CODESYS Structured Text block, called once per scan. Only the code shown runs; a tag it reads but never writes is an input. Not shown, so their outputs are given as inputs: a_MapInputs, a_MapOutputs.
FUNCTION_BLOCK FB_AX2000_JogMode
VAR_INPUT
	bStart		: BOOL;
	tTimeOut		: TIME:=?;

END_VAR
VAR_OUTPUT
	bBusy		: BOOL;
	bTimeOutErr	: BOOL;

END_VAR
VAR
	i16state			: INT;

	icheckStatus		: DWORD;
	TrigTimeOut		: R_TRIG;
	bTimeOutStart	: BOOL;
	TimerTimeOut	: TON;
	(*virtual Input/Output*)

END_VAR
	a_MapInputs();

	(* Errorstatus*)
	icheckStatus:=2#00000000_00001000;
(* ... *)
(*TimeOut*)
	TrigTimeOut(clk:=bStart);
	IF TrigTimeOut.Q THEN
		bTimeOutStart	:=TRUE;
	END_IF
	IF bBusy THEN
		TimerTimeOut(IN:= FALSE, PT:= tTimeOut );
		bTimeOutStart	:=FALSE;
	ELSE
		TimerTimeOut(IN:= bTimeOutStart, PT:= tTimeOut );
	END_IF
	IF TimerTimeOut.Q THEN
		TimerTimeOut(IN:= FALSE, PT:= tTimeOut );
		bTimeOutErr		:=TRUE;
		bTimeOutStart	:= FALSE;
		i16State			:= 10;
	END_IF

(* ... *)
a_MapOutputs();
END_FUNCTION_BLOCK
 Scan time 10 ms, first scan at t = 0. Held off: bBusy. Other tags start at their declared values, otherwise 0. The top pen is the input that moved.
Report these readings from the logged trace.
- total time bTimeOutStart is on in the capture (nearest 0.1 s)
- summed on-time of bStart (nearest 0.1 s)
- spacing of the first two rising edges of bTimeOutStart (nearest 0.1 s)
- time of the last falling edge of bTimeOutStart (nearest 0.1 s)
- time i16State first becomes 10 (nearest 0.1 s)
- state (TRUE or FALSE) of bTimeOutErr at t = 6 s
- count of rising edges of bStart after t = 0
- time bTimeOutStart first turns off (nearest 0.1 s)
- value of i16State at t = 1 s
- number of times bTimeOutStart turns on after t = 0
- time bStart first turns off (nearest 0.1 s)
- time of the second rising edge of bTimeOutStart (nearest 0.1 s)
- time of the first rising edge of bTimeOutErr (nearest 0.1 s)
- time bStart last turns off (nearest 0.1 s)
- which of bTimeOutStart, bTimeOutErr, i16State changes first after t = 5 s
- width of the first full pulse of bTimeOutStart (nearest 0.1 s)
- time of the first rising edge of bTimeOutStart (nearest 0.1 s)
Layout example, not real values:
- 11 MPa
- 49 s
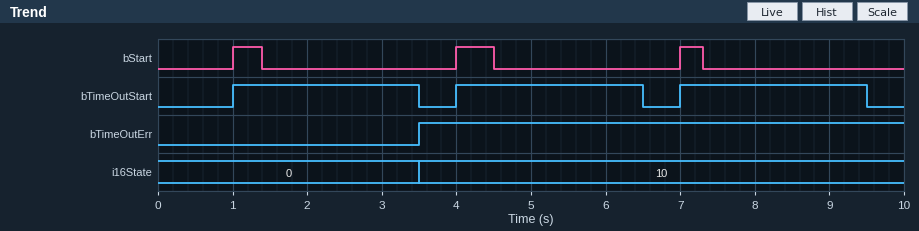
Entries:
- 7.5 s
- 1.2 s
- 3.0 s
- 9.5 s
- 3.5 s
- TRUE
- 3
- 3.5 s
- 0
- 3
- 1.4 s
- 4.0 s
- 3.5 s
- 7.3 s
- bTimeOutStart
- 2.5 s
- 1.0 s
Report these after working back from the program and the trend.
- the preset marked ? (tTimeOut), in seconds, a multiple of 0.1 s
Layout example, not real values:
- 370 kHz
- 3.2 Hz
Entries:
- 2.5 s
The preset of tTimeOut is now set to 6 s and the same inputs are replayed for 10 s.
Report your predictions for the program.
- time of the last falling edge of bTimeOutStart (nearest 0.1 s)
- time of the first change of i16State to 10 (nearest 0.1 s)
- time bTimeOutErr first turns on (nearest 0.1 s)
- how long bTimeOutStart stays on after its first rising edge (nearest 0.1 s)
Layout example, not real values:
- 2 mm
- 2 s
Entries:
- 7.0 s
- 7.0 s
- 7.0 s
- 6.0 s
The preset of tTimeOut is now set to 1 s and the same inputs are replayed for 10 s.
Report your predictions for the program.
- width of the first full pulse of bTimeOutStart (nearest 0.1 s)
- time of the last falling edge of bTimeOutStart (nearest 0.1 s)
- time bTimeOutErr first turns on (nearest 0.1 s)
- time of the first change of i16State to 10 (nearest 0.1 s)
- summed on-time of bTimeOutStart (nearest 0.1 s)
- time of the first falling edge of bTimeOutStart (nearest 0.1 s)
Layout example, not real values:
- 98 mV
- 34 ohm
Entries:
- 1.0 s
- 8.0 s
- 2.0 s
- 2.0 s
- 3.0 s
- 2.0 s
